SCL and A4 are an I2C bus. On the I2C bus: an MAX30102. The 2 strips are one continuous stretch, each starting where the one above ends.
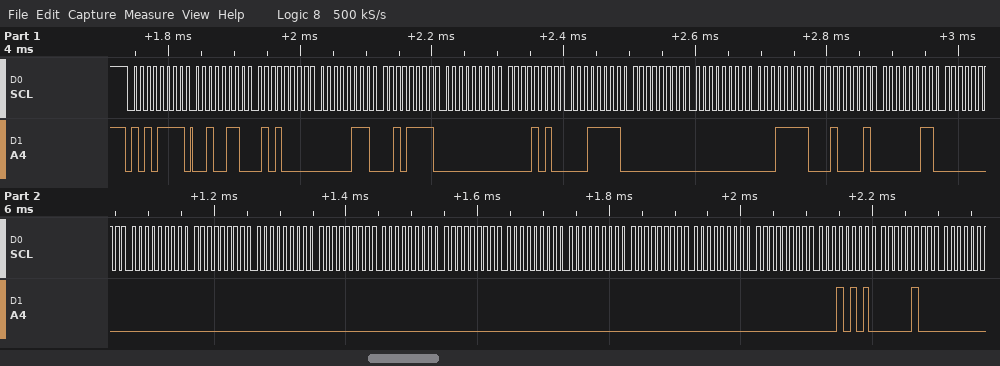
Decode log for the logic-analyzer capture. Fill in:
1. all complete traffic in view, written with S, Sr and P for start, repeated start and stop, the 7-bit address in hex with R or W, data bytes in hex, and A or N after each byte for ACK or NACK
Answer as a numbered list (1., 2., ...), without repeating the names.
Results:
1. S 57R A 26 A 50 A 07 A 2F A 00 A 0A A 1F A 00 A 00 A 1F A 21 A 03 A 00 A 00 A 00 A 00 A 00 A 00 A 00 A 00 A 00 A 00 A 00 A 00 A 15 A 04 A
